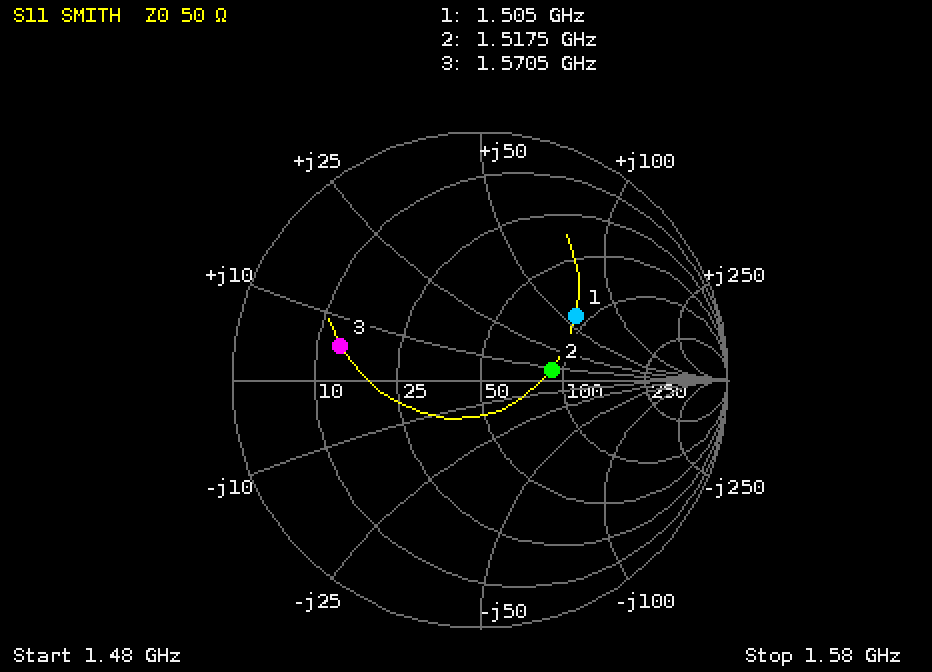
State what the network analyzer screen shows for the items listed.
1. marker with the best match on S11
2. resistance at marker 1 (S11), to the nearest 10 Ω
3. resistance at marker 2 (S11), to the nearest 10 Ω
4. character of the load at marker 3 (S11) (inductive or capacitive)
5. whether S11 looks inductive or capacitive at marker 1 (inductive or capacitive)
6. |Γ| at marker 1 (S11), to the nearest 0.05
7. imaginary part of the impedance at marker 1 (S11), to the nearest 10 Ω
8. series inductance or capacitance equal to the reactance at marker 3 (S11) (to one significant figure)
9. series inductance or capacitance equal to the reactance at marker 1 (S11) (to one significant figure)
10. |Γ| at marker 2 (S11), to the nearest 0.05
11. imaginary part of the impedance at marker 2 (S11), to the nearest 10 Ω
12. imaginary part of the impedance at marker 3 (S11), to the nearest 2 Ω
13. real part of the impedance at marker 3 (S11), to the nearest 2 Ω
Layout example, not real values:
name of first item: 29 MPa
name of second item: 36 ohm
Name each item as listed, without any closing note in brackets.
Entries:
marker with the best match on S11: marker 2
resistance at marker 1 (S11), to the nearest 10 Ω: 90 Ω
resistance at marker 2 (S11), to the nearest 10 Ω: 90 Ω
character of the load at marker 3 (S11): inductive
whether S11 looks inductive or capacitive at marker 1: inductive
|Γ| at marker 1 (S11), to the nearest 0.05: 0.45
imaginary part of the impedance at marker 1 (S11), to the nearest 10 Ω: +60 Ω
series inductance or capacitance equal to the reactance at marker 3 (S11): 600 pH
series inductance or capacitance equal to the reactance at marker 1 (S11): 6 nH
|Γ| at marker 2 (S11), to the nearest 0.05: 0.30
imaginary part of the impedance at marker 2 (S11), to the nearest 10 Ω: +10 Ω
imaginary part of the impedance at marker 3 (S11), to the nearest 2 Ω: +6 Ω
real part of the impedance at marker 3 (S11), to the nearest 2 Ω: 14 Ω
